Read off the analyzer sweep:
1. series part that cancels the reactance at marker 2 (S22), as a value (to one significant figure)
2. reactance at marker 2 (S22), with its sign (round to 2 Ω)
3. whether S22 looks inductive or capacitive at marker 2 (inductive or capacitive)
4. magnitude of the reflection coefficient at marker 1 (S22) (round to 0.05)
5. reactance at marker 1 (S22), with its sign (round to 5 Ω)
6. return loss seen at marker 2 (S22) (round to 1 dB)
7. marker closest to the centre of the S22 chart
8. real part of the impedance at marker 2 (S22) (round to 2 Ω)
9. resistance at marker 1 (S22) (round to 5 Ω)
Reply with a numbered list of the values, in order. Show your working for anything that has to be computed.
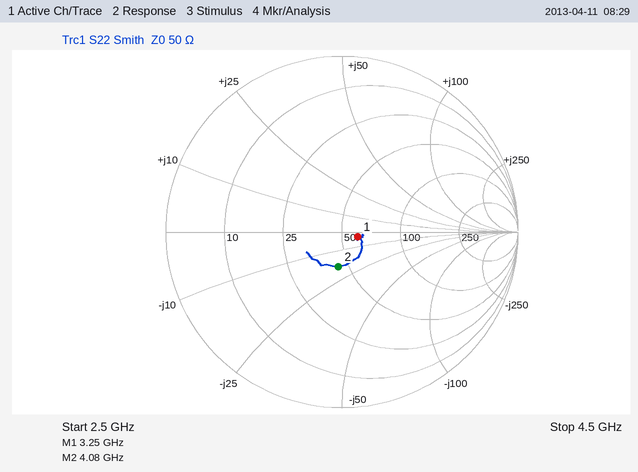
1. L = 18 Ω/(2π × 4.08 GHz) ≈ 702 pH, so 700 pH to one significant figure
2. -18 Ω
3. capacitive
4. 0.10
5. -5 Ω
6. 14 dB
7. marker 1
8. 44 Ω
9. 60 Ω
